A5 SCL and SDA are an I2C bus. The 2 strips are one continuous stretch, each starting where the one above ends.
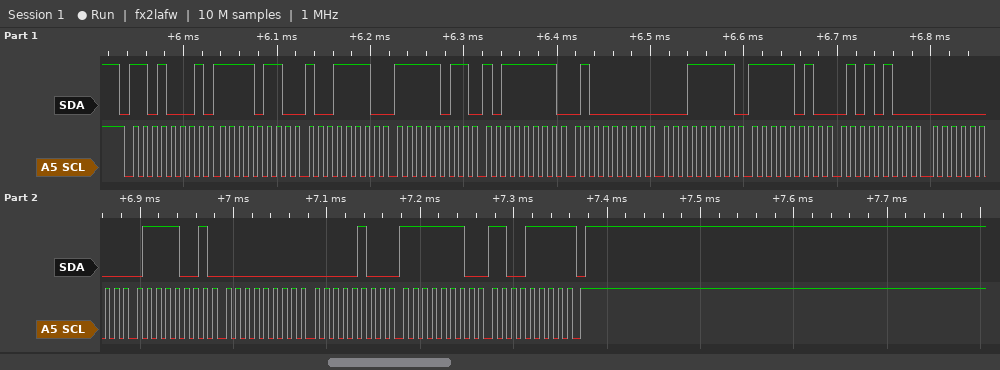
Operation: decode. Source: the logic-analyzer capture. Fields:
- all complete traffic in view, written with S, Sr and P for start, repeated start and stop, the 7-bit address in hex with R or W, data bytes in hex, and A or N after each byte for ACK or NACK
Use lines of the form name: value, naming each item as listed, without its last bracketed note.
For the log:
all complete traffic in view, written with S, Sr and P for start, repeated start and stop, the 7-bit address in hex with R or W, data bytes in hex, and A or N after each byte for ACK or NACK: S 68R A F6 A 9E A FB A BF A 40 A 1F A FA A 54 A 00 A 79 A 00 A 04 A FE A CF N P
